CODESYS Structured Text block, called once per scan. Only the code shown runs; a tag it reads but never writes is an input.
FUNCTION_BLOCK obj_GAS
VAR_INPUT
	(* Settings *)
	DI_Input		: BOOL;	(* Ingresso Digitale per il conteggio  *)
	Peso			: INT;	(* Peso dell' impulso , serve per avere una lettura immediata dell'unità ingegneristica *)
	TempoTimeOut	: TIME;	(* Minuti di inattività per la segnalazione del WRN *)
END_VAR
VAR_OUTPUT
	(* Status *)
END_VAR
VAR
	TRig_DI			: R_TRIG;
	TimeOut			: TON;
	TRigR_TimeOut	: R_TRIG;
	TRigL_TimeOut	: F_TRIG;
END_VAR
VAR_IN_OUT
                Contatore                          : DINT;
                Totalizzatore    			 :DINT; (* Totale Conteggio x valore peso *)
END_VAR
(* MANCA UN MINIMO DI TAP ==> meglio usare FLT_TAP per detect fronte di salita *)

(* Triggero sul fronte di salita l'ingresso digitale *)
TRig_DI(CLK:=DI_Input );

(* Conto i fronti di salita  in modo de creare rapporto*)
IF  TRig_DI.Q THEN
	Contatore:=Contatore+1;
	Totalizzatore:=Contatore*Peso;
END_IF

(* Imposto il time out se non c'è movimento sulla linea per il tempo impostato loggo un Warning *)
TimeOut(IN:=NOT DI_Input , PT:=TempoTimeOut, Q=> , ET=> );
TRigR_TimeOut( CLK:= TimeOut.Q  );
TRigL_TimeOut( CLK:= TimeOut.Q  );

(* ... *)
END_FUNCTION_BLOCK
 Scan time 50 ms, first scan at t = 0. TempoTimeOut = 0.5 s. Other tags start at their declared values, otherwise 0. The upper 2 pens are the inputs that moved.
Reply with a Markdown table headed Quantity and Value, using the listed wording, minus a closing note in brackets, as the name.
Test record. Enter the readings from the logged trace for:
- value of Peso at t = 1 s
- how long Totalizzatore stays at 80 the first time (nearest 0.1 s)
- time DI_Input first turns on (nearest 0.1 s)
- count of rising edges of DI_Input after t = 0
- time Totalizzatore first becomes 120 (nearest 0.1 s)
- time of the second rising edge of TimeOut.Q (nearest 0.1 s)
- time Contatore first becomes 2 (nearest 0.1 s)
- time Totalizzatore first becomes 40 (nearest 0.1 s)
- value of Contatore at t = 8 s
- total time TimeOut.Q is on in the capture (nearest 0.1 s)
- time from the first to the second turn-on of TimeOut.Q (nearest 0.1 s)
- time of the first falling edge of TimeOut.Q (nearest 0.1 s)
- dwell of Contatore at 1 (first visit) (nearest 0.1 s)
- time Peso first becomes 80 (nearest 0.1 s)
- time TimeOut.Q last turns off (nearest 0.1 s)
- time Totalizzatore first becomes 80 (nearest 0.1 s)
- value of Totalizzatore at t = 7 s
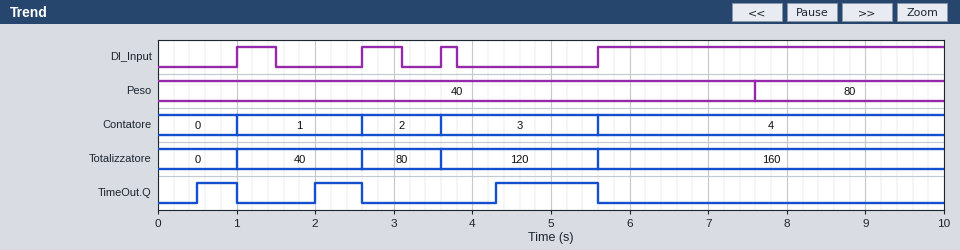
| Quantity | Value |
|---|---|
| value of Peso at t = 1 s | 40 |
| how long Totalizzatore stays at 80 the first time | 1.0 s |
| time DI_Input first turns on | 1.0 s |
| count of rising edges of DI_Input after t = 0 | 4 |
| time Totalizzatore first becomes 120 | 3.6 s |
| time of the second rising edge of TimeOut.Q | 2.0 s |
| time Contatore first becomes 2 | 2.6 s |
| time Totalizzatore first becomes 40 | 1.0 s |
| value of Contatore at t = 8 s | 4 |
| total time TimeOut.Q is on in the capture | 2.4 s |
| time from the first to the second turn-on of TimeOut.Q | 1.5 s |
| time of the first falling edge of TimeOut.Q | 1.0 s |
| dwell of Contatore at 1 (first visit) | 1.6 s |
| time Peso first becomes 80 | 7.6 s |
| time TimeOut.Q last turns off | 5.6 s |
| time Totalizzatore first becomes 80 | 2.6 s |
| value of Totalizzatore at t = 7 s | 160 |
